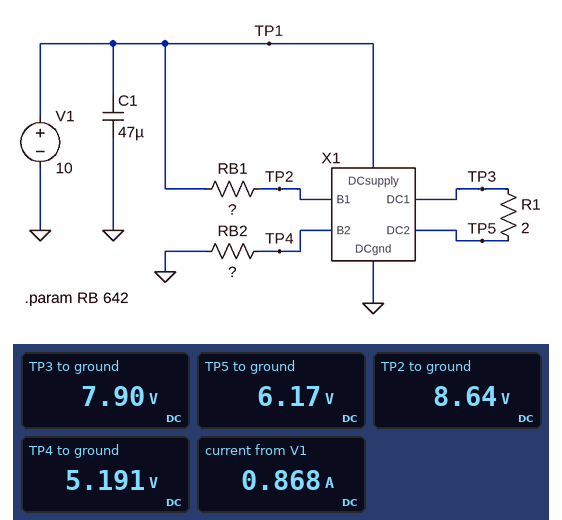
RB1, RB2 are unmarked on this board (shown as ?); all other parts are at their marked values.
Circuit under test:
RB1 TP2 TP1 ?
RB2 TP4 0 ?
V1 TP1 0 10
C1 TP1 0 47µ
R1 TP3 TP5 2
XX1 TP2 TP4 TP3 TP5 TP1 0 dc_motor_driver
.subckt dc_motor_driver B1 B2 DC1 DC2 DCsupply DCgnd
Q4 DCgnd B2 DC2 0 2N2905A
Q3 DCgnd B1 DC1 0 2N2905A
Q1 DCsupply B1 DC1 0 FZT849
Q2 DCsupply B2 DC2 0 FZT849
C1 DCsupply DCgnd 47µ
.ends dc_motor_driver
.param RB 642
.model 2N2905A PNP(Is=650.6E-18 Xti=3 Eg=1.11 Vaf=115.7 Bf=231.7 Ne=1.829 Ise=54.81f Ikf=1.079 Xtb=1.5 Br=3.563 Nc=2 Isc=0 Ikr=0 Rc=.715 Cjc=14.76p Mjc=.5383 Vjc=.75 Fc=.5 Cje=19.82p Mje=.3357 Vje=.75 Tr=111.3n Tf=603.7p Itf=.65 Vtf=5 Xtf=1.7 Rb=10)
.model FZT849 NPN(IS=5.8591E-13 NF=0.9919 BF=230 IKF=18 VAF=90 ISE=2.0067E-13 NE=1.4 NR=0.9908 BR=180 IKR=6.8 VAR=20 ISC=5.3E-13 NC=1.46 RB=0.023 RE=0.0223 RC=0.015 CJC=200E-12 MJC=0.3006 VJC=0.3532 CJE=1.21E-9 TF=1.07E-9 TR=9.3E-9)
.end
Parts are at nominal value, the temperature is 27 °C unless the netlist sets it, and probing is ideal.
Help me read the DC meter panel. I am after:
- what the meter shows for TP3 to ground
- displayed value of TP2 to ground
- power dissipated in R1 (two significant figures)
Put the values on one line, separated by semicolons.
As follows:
7.90 V; 8.64 V; 1.5 W
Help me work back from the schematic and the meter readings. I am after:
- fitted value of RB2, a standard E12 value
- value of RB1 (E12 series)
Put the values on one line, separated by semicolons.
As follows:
820 Ω; 330 Ω
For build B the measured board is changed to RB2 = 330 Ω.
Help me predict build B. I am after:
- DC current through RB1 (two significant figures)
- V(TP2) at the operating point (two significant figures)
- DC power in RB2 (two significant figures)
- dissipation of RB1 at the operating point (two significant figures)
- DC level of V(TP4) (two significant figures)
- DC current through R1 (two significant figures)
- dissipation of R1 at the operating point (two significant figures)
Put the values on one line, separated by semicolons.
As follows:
6.0 mA; 8.0 V; 41 mW; 12 mW; 3.7 V; 1.3 A; 3.2 W
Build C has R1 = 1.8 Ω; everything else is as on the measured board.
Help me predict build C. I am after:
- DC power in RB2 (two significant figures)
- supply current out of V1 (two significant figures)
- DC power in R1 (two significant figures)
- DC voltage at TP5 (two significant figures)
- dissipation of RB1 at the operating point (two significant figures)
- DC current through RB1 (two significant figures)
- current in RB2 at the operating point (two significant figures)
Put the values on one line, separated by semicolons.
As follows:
34 mW; 880 mA; 1.4 W; 6.3 V; 5.8 mW; 4.2 mA; 6.5 mA
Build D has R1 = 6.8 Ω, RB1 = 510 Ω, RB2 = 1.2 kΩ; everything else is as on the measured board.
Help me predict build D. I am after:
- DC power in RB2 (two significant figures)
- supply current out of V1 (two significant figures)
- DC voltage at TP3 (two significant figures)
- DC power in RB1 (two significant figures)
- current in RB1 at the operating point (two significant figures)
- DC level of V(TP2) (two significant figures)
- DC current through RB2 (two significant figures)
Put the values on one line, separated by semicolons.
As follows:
11 mW; 510 mA; 8.1 V; 2.9 mW; 2.4 mA; 8.8 V; 3.1 mA
